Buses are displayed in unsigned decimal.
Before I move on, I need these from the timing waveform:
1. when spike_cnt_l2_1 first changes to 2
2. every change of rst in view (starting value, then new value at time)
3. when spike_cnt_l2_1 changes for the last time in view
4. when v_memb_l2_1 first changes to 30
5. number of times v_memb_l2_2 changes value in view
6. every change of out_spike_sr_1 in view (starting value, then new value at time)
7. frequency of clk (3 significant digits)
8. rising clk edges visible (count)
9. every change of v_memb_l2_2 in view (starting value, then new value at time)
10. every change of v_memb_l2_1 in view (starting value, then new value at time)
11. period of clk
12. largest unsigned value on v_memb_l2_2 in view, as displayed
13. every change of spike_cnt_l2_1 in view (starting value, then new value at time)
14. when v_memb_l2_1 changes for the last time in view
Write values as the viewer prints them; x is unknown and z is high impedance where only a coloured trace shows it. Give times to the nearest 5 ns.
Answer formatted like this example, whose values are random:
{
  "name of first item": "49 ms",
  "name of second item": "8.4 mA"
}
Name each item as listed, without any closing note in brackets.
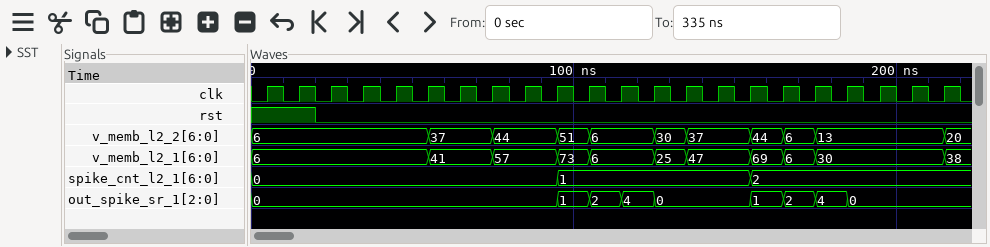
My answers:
{
  "when spike_cnt_l2_1 first changes to 2": "155 ns",
  "every change of rst in view": "1, 0 at 20 ns",
  "when spike_cnt_l2_1 changes for the last time in view": "155 ns",
  "when v_memb_l2_1 first changes to 30": "175 ns",
  "number of times v_memb_l2_2 changes value in view": "10",
  "every change of out_spike_sr_1 in view": "0, 1 at 95 ns, 2 at 105 ns, 4 at 115 ns, 0 at 125 ns, 1 at 155 ns, 2 at 165 ns, 4 at 175 ns, 0 at 185 ns",
  "frequency of clk": "100 MHz",
  "rising clk edges visible": "22",
  "every change of v_memb_l2_2 in view": "6, 37 at 55 ns, 44 at 75 ns, 51 at 95 ns, 6 at 105 ns, 30 at 125 ns, 37 at 135 ns, 44 at 155 ns, 6 at 165 ns, 13 at 175 ns, 20 at 215 ns",
  "every change of v_memb_l2_1 in view": "6, 41 at 55 ns, 57 at 75 ns, 73 at 95 ns, 6 at 105 ns, 25 at 125 ns, 47 at 135 ns, 69 at 155 ns, 6 at 165 ns, 30 at 175 ns, 38 at 215 ns",
  "period of clk": "10 ns",
  "largest unsigned value on v_memb_l2_2 in view, as displayed": "51",
  "every change of spike_cnt_l2_1 in view": "0, 1 at 95 ns, 2 at 155 ns",
  "when v_memb_l2_1 changes for the last time in view": "215 ns"
}
